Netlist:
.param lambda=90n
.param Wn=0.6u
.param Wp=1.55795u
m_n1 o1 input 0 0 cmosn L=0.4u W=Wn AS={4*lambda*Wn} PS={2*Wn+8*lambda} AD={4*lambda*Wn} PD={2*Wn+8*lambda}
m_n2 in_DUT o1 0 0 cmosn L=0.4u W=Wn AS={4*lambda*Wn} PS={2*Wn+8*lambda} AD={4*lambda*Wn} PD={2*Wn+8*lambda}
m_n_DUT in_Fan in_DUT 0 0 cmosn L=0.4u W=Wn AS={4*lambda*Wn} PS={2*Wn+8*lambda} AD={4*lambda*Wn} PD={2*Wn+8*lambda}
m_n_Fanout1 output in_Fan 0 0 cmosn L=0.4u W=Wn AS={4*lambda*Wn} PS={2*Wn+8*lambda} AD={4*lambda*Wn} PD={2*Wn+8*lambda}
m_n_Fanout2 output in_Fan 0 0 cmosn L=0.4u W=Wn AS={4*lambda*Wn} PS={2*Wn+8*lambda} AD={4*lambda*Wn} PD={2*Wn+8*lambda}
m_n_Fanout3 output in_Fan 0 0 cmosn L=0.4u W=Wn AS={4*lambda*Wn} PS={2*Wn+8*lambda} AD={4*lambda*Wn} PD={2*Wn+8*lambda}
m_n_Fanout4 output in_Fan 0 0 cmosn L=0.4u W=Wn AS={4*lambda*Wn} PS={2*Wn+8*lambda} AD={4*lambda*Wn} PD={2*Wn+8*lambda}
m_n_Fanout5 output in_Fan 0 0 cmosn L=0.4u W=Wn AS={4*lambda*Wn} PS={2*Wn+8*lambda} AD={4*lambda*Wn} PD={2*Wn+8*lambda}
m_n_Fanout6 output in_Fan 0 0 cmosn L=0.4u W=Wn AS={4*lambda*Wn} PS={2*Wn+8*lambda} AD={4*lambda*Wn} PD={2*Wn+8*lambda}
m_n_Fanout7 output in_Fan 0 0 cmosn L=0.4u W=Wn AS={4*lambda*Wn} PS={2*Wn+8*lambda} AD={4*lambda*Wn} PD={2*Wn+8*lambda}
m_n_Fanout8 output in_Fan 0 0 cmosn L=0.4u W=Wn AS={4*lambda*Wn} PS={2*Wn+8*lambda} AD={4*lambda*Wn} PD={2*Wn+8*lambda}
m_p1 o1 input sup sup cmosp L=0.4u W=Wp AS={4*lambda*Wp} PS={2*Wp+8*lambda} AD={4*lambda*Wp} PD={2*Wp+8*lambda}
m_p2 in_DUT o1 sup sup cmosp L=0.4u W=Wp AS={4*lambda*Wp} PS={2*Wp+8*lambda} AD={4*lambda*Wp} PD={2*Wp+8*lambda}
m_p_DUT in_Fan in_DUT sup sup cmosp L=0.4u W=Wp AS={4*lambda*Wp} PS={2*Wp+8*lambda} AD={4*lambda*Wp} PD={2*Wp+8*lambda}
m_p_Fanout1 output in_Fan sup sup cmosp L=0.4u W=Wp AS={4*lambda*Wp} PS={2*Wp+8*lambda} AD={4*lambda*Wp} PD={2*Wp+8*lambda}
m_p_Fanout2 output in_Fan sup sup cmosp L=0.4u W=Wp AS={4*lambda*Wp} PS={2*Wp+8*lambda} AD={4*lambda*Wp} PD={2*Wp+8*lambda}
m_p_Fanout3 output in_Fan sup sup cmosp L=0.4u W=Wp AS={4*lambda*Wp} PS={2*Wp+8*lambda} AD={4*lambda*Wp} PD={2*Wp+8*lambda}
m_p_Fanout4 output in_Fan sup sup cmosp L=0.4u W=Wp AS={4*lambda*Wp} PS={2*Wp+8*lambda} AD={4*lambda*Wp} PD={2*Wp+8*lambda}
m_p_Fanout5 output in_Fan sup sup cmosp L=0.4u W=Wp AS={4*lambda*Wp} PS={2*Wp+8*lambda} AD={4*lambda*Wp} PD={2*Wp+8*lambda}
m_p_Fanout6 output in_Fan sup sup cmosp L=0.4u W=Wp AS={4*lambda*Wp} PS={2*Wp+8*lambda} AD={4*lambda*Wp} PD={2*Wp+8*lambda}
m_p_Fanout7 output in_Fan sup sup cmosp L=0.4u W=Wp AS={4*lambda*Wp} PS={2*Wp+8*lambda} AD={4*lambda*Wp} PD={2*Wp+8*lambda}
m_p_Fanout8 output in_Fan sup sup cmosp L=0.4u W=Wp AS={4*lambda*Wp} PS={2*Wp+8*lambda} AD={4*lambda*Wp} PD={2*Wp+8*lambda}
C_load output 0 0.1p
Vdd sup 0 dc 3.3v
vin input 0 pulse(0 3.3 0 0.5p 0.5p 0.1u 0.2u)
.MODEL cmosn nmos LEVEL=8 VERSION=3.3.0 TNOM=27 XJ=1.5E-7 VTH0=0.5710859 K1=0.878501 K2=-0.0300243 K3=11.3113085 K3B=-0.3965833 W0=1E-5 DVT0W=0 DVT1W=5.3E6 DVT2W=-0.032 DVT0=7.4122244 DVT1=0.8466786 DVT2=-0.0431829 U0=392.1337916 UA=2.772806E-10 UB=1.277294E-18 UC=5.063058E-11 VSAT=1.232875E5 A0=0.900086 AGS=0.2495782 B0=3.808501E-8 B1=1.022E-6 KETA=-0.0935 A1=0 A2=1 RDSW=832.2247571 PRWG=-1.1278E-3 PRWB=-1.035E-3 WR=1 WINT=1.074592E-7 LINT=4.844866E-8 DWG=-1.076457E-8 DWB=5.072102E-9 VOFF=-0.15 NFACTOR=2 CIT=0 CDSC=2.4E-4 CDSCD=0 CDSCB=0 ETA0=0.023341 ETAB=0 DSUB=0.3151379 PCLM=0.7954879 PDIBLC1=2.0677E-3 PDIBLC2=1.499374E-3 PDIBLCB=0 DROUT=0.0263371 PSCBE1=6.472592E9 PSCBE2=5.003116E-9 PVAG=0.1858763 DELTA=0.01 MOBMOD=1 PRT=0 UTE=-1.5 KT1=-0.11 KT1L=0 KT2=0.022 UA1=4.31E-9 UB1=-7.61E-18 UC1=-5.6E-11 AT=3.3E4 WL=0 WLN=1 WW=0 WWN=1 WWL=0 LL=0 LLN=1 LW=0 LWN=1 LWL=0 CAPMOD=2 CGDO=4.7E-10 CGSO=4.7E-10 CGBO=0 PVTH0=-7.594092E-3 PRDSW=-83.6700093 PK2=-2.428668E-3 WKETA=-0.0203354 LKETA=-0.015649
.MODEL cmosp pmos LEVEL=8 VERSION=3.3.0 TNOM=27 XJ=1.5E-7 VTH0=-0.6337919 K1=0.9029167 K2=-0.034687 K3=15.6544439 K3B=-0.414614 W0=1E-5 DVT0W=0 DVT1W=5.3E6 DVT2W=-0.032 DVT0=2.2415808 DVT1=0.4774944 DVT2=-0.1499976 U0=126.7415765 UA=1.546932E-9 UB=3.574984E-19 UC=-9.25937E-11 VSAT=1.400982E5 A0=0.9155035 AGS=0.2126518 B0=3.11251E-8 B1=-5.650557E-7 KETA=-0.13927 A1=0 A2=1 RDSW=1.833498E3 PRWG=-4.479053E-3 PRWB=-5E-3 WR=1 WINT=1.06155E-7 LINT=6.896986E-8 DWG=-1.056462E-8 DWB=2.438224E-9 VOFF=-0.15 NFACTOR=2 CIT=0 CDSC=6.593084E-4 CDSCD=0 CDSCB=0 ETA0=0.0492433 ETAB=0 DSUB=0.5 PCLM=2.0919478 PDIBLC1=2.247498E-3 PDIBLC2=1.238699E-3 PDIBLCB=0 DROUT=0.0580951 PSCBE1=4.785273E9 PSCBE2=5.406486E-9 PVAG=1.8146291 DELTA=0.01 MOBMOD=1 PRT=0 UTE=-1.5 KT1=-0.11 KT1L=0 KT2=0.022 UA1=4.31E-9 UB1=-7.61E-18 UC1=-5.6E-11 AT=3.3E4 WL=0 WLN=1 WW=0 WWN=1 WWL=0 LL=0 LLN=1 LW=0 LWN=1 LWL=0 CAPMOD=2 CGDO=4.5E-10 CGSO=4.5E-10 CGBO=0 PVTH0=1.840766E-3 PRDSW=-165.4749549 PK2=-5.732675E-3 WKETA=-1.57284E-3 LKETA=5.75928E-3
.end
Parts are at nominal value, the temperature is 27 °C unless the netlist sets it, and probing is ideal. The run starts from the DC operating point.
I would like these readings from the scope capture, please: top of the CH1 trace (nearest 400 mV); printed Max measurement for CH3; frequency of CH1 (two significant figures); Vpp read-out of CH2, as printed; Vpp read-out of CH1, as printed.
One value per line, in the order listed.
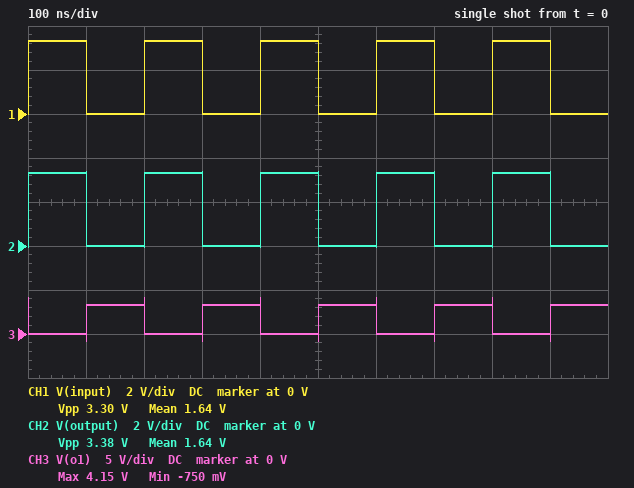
3.2 V
4.15 V
5.0 MHz
3.38 V
3.30 V
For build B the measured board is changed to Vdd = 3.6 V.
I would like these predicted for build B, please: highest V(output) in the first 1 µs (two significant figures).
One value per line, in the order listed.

3.7 V
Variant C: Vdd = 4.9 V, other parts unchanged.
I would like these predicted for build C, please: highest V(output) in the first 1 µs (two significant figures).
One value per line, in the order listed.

5.0 V
